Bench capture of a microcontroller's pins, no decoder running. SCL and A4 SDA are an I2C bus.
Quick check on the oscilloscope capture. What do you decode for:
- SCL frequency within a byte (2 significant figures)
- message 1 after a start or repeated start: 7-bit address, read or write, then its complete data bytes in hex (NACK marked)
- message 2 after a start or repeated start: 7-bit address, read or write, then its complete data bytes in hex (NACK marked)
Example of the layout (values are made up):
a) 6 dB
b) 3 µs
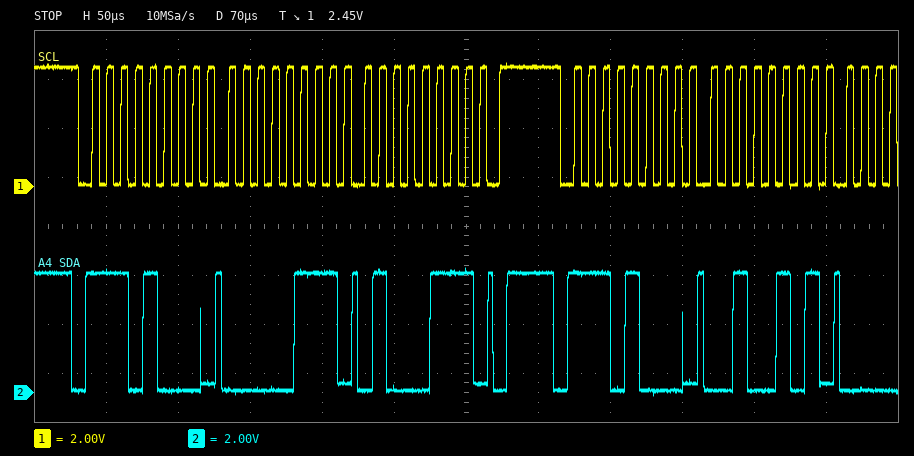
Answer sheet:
a) 100 kHz
b) 0x74 write: 07 47
c) 0x74 write: 25
